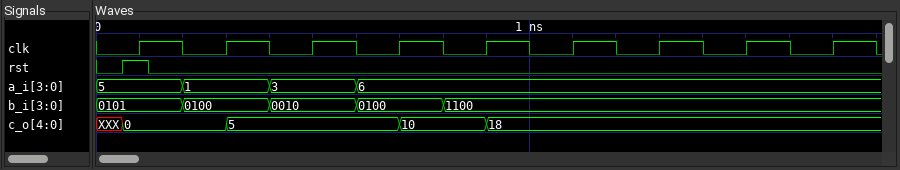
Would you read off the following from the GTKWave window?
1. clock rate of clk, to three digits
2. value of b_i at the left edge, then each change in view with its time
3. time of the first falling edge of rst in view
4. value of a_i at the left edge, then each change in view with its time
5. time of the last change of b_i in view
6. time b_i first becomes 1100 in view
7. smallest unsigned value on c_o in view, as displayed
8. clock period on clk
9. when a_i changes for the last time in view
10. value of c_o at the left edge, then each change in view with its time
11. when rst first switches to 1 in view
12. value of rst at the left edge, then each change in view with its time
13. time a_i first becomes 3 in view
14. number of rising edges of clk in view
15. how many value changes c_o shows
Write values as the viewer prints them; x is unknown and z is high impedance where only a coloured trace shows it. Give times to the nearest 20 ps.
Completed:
5.00 GHz
0101, 0100 at 200 ps, 0010 at 400 ps, 0100 at 600 ps, 1100 at 800 ps
120 ps
5, 1 at 200 ps, 3 at 400 ps, 6 at 600 ps
800 ps
800 ps
0
200 ps
600 ps
XXX, 0 at 60 ps, 5 at 300 ps, 10 at 700 ps, 18 at 900 ps
60 ps
0, 1 at 60 ps, 0 at 120 ps
400 ps
9
4
